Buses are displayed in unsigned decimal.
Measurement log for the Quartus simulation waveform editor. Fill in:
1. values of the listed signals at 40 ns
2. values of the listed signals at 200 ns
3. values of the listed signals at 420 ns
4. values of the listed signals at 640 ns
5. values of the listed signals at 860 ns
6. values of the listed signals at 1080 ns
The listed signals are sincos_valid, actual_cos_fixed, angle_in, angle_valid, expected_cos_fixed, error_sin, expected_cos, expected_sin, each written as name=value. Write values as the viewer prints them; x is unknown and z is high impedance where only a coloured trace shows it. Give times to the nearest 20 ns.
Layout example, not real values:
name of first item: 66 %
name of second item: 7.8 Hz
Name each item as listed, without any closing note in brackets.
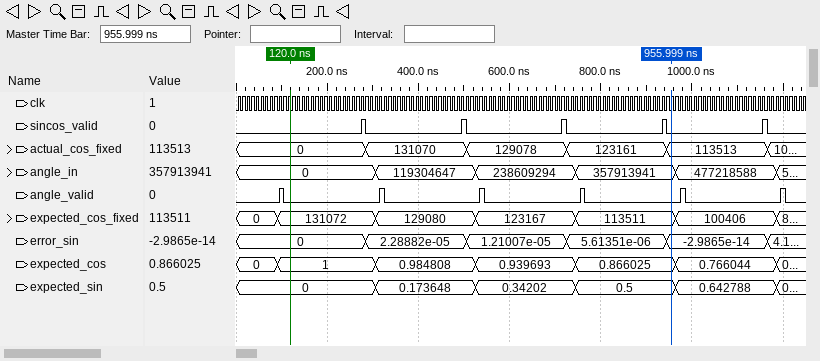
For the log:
values of the listed signals at 40 ns: sincos_valid=0, actual_cos_fixed=0, angle_in=0, angle_valid=0, expected_cos_fixed=0, error_sin=0, expected_cos=0, expected_sin=0
values of the listed signals at 200 ns: sincos_valid=0, actual_cos_fixed=0, angle_in=0, angle_valid=0, expected_cos_fixed=131072, error_sin=0, expected_cos=1, expected_sin=0
values of the listed signals at 420 ns: sincos_valid=0, actual_cos_fixed=131070, angle_in=119304647, angle_valid=0, expected_cos_fixed=129080, error_sin=2.28882e-05, expected_cos=0.984808, expected_sin=0.173648
values of the listed signals at 640 ns: sincos_valid=0, actual_cos_fixed=129078, angle_in=238609294, angle_valid=0, expected_cos_fixed=123167, error_sin=1.21007e-05, expected_cos=0.939693, expected_sin=0.34202
values of the listed signals at 860 ns: sincos_valid=0, actual_cos_fixed=123161, angle_in=357913941, angle_valid=0, expected_cos_fixed=113511, error_sin=5.61351e-06, expected_cos=0.866025, expected_sin=0.5
values of the listed signals at 1080 ns: sincos_valid=0, actual_cos_fixed=113513, angle_in=477218588, angle_valid=0, expected_cos_fixed=100406, error_sin=-2.9865e-14, expected_cos=0.766044, expected_sin=0.642788
